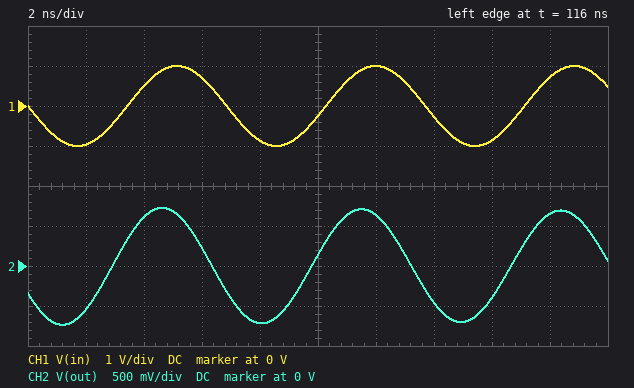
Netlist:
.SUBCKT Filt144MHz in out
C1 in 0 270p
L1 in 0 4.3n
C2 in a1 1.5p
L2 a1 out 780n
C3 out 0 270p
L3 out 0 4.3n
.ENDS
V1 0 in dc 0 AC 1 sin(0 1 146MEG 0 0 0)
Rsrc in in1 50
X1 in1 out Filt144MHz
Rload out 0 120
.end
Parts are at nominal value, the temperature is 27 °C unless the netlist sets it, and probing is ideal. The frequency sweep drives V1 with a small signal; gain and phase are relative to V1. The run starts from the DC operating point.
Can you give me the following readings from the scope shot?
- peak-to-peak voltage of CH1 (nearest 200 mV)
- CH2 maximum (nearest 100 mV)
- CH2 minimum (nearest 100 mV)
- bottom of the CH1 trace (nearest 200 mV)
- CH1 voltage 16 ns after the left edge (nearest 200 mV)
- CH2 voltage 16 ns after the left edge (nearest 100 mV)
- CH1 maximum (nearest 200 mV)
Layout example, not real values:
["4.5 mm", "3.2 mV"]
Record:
["2.0 V", "700 mV", "-700 mV", "-1.0 V", "-800 mV", "-400 mV", "1.0 V"]
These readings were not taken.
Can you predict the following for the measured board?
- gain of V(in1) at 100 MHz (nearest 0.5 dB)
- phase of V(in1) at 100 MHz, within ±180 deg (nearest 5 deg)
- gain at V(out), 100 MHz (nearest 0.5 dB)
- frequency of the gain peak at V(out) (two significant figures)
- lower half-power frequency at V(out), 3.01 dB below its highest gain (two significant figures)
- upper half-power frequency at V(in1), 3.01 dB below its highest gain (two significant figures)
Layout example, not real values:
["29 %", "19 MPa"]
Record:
["-20.0 dB", "-95 deg", "-61.0 dB", "150 MHz", "140 MHz", "160 MHz"]
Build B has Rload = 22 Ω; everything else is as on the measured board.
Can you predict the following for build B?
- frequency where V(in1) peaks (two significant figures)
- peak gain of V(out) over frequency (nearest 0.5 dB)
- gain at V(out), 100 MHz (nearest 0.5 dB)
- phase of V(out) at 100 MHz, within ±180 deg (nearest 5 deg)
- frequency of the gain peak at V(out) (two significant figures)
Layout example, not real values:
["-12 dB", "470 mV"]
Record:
["150 MHz", "-10.0 dB", "-61.5 dB", "70 deg", "140 MHz"]
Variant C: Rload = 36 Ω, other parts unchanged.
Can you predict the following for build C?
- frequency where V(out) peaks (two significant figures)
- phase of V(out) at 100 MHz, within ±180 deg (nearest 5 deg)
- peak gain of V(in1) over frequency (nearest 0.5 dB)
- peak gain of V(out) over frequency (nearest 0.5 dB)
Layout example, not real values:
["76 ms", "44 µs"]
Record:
["140 MHz", "75 deg", "-2.5 dB", "-7.5 dB"]
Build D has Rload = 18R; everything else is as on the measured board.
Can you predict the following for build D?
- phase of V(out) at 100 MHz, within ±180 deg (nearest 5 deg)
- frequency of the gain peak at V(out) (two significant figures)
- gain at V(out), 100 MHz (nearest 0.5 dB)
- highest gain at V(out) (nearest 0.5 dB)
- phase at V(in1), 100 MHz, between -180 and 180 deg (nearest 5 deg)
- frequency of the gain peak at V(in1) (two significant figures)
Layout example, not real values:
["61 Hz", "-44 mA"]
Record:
["70 deg", "140 MHz", "-61.5 dB", "-11.0 dB", "-95 deg", "150 MHz"]
